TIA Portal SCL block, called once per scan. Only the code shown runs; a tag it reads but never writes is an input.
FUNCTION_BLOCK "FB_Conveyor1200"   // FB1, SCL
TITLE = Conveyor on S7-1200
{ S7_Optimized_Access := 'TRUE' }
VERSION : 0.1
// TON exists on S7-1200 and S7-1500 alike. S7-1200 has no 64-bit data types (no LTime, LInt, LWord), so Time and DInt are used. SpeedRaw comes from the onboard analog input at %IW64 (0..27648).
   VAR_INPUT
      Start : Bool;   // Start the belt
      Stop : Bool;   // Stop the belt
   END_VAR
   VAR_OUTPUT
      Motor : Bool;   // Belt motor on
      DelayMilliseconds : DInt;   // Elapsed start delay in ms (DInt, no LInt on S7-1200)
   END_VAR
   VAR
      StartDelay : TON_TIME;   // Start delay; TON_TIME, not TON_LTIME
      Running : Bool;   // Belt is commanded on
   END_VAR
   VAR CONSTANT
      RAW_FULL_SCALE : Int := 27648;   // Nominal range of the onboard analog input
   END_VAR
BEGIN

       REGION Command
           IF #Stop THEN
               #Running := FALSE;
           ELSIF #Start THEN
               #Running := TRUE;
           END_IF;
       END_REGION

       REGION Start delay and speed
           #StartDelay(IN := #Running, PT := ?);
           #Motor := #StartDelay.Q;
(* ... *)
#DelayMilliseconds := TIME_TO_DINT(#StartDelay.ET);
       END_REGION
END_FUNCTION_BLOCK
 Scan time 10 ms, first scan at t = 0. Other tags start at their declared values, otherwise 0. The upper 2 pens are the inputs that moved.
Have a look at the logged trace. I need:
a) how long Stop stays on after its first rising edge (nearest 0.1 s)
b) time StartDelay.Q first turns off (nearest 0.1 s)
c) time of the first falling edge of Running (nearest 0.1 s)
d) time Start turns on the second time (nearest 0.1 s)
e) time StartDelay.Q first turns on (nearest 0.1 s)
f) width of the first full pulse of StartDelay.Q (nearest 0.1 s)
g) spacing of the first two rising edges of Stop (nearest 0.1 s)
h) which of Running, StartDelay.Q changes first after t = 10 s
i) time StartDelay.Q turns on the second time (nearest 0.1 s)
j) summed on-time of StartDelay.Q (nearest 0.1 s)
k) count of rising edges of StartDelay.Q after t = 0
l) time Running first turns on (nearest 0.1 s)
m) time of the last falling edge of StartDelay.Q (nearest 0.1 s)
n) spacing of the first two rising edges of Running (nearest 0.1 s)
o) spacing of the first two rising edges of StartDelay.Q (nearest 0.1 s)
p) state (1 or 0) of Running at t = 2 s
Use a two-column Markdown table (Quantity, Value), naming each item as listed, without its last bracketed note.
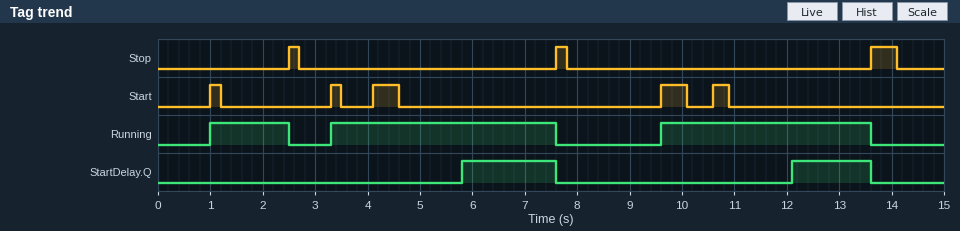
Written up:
| Quantity | Value |
|---|---|
| how long Stop stays on after its first rising edge | 0.2 s |
| time StartDelay.Q first turns off | 7.6 s |
| time of the first falling edge of Running | 2.5 s |
| time Start turns on the second time | 3.3 s |
| time StartDelay.Q first turns on | 5.8 s |
| width of the first full pulse of StartDelay.Q | 1.8 s |
| spacing of the first two rising edges of Stop | 5.1 s |
| which of Running, StartDelay.Q changes first after t = 10 s | StartDelay.Q |
| time StartDelay.Q turns on the second time | 12.1 s |
| summed on-time of StartDelay.Q | 3.3 s |
| count of rising edges of StartDelay.Q after t = 0 | 2 |
| time Running first turns on | 1.0 s |
| time of the last falling edge of StartDelay.Q | 13.6 s |
| spacing of the first two rising edges of Running | 2.3 s |
| spacing of the first two rising edges of StartDelay.Q | 6.3 s |
| state (1 or 0) of Running at t = 2 s | 1 |
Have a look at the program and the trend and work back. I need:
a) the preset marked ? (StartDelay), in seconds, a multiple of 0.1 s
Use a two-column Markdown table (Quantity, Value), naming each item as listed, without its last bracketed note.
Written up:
| Quantity | Value |
|---|---|
| the preset marked ? (StartDelay), in seconds, a multiple of 0.1 s | 2.5 s |
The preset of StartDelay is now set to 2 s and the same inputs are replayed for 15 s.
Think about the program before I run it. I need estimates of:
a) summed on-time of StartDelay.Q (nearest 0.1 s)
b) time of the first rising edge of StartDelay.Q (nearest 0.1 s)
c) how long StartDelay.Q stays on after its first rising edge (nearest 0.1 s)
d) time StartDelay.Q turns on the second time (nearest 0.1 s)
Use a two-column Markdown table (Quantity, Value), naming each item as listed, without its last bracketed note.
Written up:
| Quantity | Value |
|---|---|
| summed on-time of StartDelay.Q | 4.3 s |
| time of the first rising edge of StartDelay.Q | 5.3 s |
| how long StartDelay.Q stays on after its first rising edge | 2.3 s |
| time StartDelay.Q turns on the second time | 11.6 s |
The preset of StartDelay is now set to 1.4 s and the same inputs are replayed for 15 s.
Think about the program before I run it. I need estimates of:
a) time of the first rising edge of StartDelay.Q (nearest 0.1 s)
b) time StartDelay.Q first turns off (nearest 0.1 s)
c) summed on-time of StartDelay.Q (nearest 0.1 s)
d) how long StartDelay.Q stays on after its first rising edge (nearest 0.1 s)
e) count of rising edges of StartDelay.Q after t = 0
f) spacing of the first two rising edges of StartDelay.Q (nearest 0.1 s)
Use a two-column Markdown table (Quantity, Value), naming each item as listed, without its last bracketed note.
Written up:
| Quantity | Value |
|---|---|
| time of the first rising edge of StartDelay.Q | 2.4 s |
| time StartDelay.Q first turns off | 2.5 s |
| summed on-time of StartDelay.Q | 5.6 s |
| how long StartDelay.Q stays on after its first rising edge | 0.1 s |
| count of rising edges of StartDelay.Q after t = 0 | 3 |
| spacing of the first two rising edges of StartDelay.Q | 2.3 s |
